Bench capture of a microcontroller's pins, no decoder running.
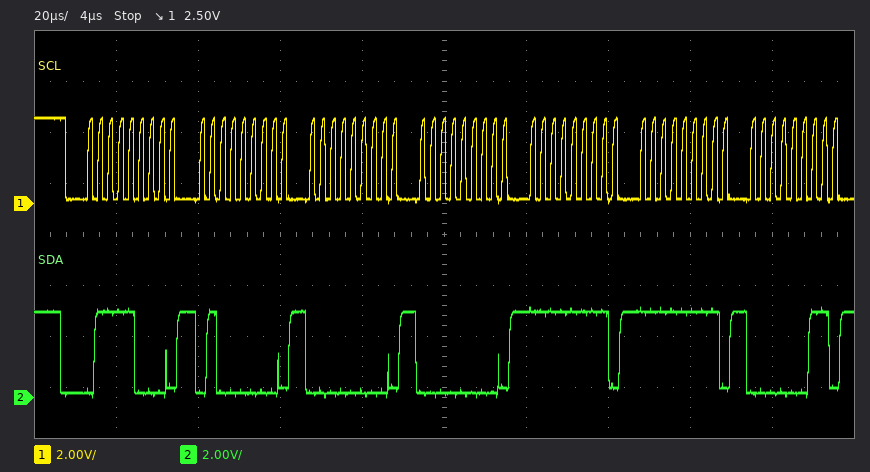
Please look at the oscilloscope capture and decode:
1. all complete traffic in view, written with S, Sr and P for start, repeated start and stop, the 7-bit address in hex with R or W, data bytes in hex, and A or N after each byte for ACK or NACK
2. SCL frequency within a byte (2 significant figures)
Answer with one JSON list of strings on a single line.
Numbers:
["S 3CW A 40 A 00 A 00 A FF A FF A 03 A", "400 kHz"]
